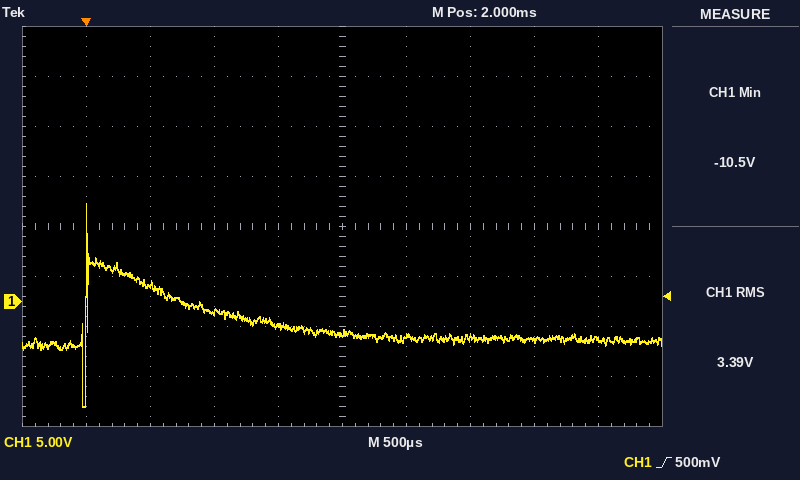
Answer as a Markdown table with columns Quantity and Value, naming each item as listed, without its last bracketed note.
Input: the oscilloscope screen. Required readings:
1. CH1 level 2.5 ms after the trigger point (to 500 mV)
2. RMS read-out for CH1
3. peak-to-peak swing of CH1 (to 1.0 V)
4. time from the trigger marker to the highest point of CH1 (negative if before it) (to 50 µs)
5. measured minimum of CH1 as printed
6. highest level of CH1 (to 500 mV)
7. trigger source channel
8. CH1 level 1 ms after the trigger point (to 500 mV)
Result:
| Quantity | Value |
|---|---|
| CH1 level 2.5 ms after the trigger point | -3.5 V |
| RMS read-out for CH1 | 3.39 V |
| peak-to-peak swing of CH1 | 20.0 V |
| time from the trigger marker to the highest point of CH1 (negative if before it) | 0 µs |
| measured minimum of CH1 as printed | -10.5 V |
| highest level of CH1 | 10.0 V |
| trigger source channel | CH1 |
| CH1 level 1 ms after the trigger point | -1.0 V |
